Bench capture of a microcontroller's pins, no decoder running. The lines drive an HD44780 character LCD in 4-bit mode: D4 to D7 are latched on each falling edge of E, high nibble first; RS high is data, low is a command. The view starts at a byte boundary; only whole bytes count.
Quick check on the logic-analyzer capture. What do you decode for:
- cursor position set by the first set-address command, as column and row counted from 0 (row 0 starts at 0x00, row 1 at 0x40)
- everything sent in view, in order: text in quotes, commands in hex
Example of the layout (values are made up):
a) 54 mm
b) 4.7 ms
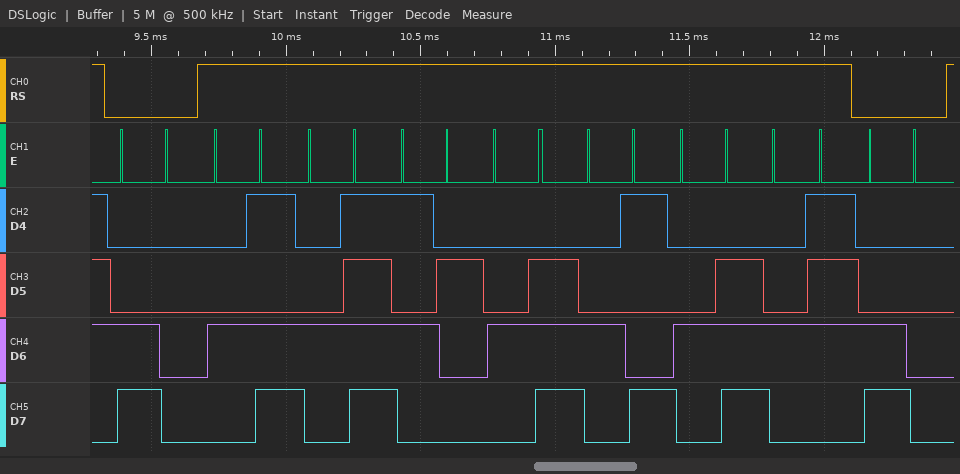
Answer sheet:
a) column 0, row 1
b) 0xC0 "MORNING" 0xC0
